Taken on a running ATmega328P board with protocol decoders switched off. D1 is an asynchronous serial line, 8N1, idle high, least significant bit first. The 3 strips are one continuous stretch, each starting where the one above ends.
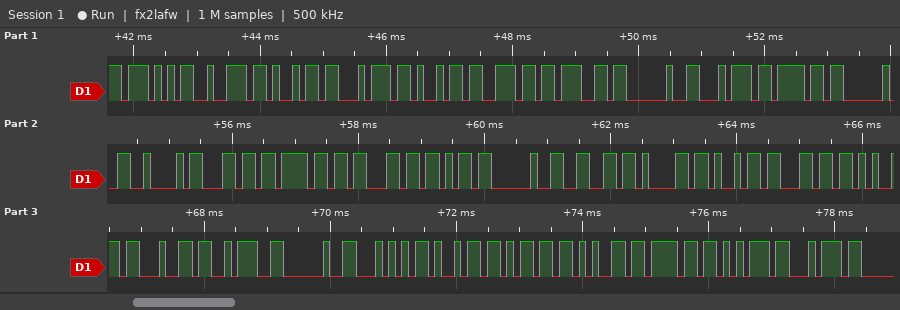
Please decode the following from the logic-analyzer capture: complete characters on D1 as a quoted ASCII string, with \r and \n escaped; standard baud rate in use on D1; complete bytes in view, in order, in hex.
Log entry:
"Writing to Block failed: Timeout"
9600 baud
0x57 0x72 0x69 0x74 0x69 0x6E 0x67 0x20 0x74 0x6F 0x20 0x42 0x6C 0x6F 0x63 0x6B 0x20 0x66 0x61 0x69 0x6C 0x65 0x64 0x3A 0x20 0x54 0x69 0x6D 0x65 0x6F 0x75 0x74
